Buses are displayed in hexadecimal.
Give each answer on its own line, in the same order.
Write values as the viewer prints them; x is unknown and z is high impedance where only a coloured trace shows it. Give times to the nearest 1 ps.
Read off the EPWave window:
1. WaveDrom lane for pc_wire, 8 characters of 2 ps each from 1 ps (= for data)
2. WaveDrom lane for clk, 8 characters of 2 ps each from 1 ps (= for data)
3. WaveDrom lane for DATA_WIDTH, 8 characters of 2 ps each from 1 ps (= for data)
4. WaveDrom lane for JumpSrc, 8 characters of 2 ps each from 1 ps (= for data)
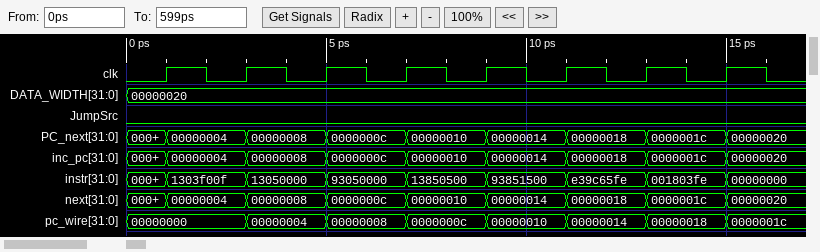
{name: 'pc_wire', wave: '========', data: '00000000 00000004 00000008 0000000c 00000010 00000014 00000018 0000001c'}
{name: 'clk', wave: 'p.......'}
{name: 'DATA_WIDTH', wave: '=.......', data: '00000020'}
{name: 'JumpSrc', wave: '0.......'}
